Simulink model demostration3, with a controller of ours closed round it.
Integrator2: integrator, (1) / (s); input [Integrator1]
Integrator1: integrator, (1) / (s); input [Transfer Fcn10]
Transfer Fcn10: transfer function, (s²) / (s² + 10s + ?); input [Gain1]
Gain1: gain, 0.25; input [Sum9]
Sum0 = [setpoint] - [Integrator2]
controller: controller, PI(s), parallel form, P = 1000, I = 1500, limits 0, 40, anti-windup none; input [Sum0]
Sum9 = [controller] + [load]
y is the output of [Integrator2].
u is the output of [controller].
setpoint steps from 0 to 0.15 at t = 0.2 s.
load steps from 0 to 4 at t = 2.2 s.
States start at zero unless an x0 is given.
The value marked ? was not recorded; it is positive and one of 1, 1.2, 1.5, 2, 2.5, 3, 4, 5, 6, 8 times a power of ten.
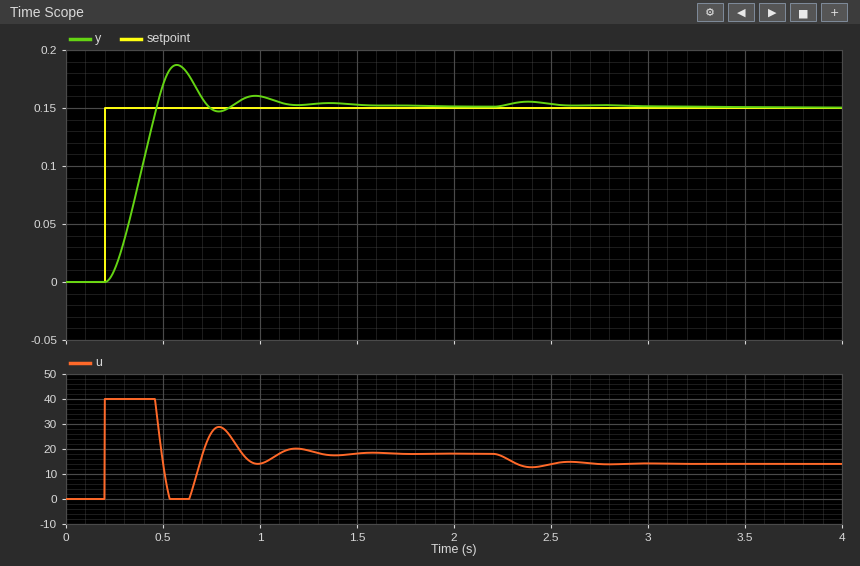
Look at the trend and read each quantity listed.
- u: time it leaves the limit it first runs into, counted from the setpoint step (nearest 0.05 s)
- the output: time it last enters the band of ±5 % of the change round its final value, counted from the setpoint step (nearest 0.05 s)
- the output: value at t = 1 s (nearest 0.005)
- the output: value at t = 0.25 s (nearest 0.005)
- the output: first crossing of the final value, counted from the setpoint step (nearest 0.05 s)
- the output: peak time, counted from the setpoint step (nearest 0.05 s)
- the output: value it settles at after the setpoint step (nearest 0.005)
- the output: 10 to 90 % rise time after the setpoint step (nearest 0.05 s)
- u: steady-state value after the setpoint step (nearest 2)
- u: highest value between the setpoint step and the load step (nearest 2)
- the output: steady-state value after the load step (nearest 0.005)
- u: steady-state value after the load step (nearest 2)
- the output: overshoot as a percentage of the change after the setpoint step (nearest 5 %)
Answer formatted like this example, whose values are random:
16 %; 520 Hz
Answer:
0.25 s; 0.85 s; 0.160; 0.010; 0.25 s; 0.35 s; 0.150; 0.20 s; 18; 40; 0.150; 14; 25 %
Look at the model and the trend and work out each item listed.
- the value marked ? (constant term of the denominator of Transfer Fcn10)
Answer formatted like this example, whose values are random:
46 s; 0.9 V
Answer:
30
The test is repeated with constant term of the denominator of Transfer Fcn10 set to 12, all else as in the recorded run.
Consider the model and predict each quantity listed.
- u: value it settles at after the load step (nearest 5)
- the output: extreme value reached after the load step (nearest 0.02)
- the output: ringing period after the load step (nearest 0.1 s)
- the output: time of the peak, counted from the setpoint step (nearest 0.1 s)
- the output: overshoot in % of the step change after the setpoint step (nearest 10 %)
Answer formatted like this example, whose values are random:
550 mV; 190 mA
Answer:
5; 0.16; 0.4 s; 0.4 s; 40 %
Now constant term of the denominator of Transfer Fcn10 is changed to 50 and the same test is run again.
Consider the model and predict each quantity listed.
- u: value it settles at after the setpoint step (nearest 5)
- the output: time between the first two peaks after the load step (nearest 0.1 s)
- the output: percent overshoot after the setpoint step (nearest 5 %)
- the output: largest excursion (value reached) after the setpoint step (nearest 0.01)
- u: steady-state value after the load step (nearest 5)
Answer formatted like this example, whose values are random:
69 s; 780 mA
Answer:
30; 0.4 s; 15 %; 0.17; 25
